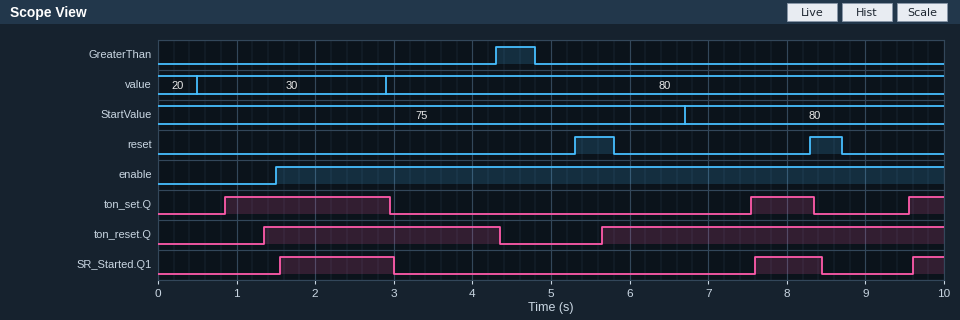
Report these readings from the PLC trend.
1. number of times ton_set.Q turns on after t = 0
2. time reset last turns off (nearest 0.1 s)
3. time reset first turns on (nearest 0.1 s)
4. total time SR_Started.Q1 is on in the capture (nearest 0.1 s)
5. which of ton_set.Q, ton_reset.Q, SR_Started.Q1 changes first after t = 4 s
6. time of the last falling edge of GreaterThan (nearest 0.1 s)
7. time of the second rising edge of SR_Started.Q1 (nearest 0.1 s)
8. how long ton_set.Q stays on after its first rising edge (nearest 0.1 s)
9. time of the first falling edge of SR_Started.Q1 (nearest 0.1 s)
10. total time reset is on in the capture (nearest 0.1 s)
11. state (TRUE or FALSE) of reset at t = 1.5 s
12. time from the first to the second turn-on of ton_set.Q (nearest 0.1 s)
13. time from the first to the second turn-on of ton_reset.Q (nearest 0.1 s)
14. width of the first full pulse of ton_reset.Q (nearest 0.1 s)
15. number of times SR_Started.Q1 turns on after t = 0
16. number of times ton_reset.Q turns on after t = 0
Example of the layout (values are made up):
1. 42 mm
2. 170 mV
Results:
1. 3
2. 8.7 s
3. 5.3 s
4. 2.7 s
5. ton_reset.Q
6. 4.8 s
7. 7.6 s
8. 2.1 s
9. 3.0 s
10. 0.9 s
11. FALSE
12. 6.7 s
13. 4.3 s
14. 3.0 s
15. 3
16. 2
